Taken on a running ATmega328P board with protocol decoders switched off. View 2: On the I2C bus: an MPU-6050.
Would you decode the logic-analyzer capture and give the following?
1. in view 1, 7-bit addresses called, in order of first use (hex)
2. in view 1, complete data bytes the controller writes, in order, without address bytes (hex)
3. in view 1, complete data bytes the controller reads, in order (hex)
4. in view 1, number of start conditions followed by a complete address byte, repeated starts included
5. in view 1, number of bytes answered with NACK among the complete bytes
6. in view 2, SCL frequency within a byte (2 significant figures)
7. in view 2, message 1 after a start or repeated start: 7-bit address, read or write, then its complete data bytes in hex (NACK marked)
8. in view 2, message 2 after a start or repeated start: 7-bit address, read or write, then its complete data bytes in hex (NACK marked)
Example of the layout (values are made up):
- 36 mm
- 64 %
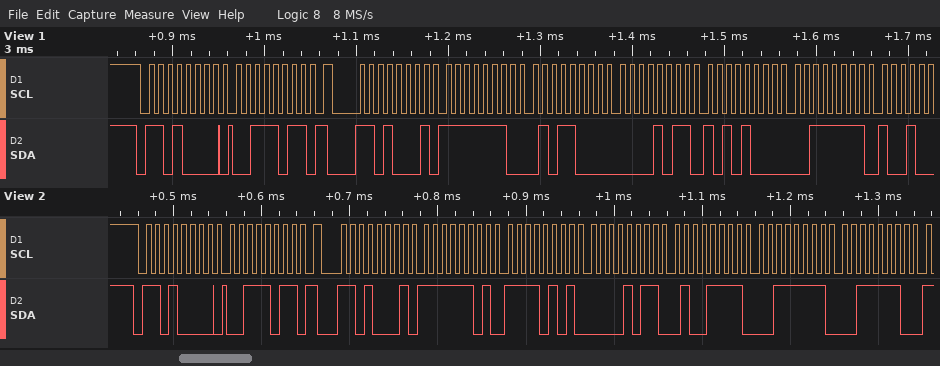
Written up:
- 0x68
- 3B
- FE 58 0B A8 3F
- 2
- 0
- 100 kHz
- 0x68 write: 3B
- 0x68 read: FD F5 0B 4F 3F 3E
